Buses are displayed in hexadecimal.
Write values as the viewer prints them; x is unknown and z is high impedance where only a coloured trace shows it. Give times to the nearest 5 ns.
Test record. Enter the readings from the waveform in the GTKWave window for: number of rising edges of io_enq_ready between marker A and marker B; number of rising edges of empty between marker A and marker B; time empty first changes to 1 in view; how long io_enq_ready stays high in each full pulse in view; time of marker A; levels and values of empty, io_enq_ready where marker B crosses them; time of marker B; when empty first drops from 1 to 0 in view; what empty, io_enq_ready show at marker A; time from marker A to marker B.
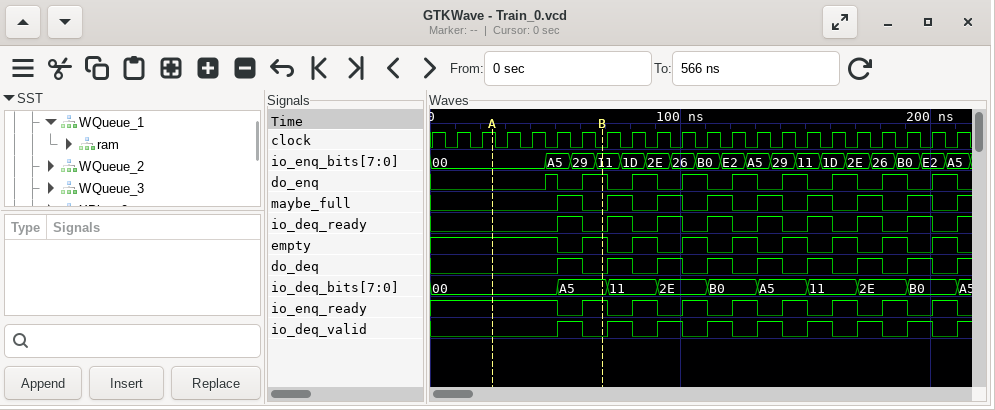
1
1
60 ns
10 ns, 10 ns, 10 ns, 10 ns, 10 ns, 10 ns, 10 ns, 10 ns
25 ns
empty=1, io_enq_ready=1
70 ns
50 ns
empty=1, io_enq_ready=1
45 ns
